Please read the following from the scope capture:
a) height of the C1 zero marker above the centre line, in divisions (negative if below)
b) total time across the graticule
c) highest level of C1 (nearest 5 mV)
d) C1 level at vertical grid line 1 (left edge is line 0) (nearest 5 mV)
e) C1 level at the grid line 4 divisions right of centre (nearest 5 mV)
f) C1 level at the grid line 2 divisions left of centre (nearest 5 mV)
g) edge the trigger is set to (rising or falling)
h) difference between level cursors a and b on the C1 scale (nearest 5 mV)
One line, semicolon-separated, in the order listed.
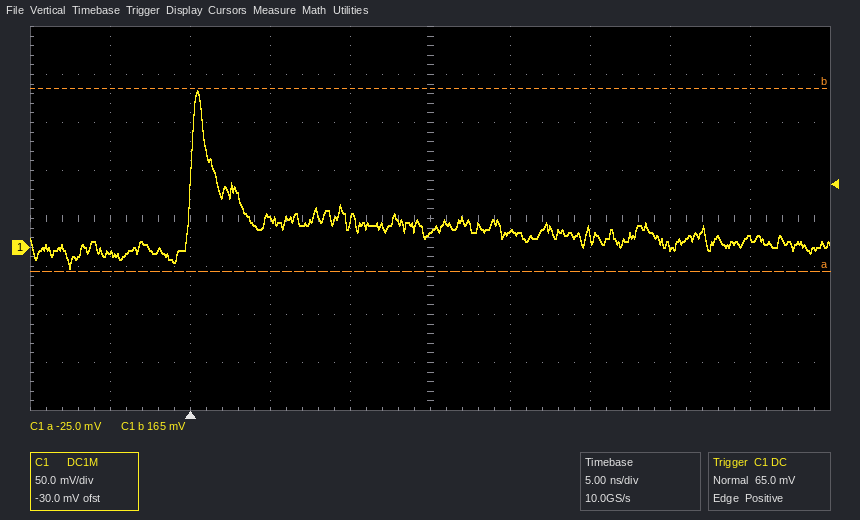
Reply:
-0.6 div; 50 ns; 165 mV; -5 mV; 10 mV; 30 mV; rising; 190 mV
